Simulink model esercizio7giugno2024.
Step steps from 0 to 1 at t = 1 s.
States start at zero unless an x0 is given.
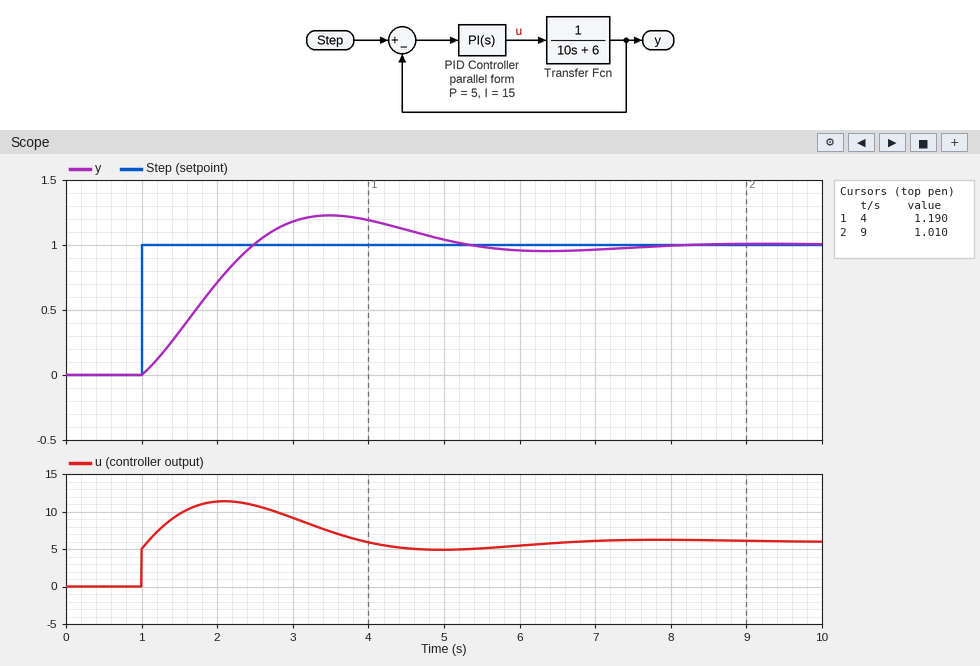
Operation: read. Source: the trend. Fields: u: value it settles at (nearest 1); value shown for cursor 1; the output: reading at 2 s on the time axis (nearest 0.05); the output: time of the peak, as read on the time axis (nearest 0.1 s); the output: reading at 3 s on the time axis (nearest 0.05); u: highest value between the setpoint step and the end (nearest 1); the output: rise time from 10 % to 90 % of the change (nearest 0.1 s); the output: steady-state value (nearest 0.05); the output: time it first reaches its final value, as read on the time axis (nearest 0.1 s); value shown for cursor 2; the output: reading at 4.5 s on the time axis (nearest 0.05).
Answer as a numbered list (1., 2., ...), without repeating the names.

1. 6
2. 1.190
3. 0.70
4. 3.5 s
5. 1.20
6. 11
7. 1.1 s
8. 1.00
9. 2.5 s
10. 1.010
11. 1.10
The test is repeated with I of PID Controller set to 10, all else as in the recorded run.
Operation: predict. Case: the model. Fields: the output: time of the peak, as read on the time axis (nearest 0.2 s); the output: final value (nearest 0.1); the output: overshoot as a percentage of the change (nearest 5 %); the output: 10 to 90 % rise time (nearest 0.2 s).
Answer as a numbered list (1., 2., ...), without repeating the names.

1. 4.2 s
2. 1.0
3. 15 %
4. 1.4 s
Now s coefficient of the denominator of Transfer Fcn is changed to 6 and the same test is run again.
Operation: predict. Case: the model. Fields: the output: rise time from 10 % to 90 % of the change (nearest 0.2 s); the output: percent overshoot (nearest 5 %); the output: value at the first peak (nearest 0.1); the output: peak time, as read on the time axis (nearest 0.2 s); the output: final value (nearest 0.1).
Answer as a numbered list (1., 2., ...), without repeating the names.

1. 1.0 s
2. 15 %
3. 1.1
4. 3.0 s
5. 1.0
